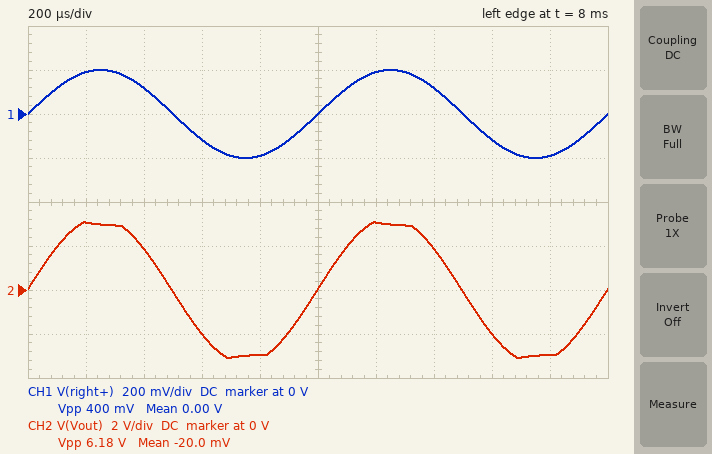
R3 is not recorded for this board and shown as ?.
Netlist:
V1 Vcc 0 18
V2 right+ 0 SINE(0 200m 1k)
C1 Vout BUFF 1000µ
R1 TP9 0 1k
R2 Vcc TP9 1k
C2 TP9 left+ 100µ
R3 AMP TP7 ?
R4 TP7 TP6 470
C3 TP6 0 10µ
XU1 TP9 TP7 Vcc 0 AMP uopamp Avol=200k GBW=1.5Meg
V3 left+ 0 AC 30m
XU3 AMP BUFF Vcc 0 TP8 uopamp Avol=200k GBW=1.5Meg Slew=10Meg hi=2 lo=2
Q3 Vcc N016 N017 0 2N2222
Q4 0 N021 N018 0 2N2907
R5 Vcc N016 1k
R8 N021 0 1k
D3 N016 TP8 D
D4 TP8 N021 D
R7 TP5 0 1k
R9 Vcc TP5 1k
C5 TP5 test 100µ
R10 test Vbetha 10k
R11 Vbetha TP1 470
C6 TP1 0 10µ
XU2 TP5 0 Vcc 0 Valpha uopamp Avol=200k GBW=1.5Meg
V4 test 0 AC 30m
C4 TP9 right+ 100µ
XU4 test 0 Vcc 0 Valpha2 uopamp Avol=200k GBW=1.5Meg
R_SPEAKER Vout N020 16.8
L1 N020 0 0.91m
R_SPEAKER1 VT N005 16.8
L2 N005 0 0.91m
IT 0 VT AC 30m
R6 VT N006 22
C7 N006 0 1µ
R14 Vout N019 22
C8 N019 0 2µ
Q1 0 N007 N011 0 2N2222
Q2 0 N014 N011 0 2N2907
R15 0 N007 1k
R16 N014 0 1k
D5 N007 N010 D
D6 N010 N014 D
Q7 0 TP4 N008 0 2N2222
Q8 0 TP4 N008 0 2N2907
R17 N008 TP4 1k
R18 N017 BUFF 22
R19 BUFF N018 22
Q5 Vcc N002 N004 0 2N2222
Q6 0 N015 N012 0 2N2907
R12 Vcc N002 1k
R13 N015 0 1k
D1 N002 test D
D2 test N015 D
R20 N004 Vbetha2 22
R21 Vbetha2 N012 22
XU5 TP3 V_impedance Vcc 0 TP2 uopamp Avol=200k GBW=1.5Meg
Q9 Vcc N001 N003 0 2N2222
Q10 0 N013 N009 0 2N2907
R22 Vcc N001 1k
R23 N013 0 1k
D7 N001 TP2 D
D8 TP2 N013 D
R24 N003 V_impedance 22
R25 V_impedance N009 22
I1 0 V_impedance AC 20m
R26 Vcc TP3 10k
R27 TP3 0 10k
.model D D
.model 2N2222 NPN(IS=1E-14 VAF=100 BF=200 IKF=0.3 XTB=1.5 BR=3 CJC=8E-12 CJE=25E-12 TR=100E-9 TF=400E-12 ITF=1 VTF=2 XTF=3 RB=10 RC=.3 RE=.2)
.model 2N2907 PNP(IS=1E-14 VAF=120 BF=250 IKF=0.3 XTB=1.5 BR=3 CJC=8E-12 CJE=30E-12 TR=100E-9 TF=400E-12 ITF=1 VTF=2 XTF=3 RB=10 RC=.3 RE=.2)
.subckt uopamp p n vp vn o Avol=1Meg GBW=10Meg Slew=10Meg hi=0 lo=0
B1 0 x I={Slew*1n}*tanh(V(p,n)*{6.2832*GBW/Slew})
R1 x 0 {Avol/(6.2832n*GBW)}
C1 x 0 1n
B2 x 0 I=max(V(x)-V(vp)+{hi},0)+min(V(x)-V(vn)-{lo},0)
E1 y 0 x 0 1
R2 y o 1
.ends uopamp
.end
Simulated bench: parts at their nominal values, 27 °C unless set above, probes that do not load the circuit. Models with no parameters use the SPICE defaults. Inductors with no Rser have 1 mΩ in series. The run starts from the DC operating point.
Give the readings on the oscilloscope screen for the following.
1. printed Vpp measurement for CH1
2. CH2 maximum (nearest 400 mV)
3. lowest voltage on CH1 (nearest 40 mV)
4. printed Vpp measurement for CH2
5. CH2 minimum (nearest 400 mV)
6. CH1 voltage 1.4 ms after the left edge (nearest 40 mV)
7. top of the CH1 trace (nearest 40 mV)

400 mV
3.2 V
-200 mV
6.18 V
-3.2 V
120 mV
200 mV
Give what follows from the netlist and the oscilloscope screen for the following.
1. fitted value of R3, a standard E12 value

15 kΩ
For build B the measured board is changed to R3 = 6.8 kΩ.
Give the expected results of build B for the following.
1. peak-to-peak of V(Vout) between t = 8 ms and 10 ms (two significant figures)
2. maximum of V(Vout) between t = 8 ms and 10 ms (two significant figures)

3.1 V
1.5 V
